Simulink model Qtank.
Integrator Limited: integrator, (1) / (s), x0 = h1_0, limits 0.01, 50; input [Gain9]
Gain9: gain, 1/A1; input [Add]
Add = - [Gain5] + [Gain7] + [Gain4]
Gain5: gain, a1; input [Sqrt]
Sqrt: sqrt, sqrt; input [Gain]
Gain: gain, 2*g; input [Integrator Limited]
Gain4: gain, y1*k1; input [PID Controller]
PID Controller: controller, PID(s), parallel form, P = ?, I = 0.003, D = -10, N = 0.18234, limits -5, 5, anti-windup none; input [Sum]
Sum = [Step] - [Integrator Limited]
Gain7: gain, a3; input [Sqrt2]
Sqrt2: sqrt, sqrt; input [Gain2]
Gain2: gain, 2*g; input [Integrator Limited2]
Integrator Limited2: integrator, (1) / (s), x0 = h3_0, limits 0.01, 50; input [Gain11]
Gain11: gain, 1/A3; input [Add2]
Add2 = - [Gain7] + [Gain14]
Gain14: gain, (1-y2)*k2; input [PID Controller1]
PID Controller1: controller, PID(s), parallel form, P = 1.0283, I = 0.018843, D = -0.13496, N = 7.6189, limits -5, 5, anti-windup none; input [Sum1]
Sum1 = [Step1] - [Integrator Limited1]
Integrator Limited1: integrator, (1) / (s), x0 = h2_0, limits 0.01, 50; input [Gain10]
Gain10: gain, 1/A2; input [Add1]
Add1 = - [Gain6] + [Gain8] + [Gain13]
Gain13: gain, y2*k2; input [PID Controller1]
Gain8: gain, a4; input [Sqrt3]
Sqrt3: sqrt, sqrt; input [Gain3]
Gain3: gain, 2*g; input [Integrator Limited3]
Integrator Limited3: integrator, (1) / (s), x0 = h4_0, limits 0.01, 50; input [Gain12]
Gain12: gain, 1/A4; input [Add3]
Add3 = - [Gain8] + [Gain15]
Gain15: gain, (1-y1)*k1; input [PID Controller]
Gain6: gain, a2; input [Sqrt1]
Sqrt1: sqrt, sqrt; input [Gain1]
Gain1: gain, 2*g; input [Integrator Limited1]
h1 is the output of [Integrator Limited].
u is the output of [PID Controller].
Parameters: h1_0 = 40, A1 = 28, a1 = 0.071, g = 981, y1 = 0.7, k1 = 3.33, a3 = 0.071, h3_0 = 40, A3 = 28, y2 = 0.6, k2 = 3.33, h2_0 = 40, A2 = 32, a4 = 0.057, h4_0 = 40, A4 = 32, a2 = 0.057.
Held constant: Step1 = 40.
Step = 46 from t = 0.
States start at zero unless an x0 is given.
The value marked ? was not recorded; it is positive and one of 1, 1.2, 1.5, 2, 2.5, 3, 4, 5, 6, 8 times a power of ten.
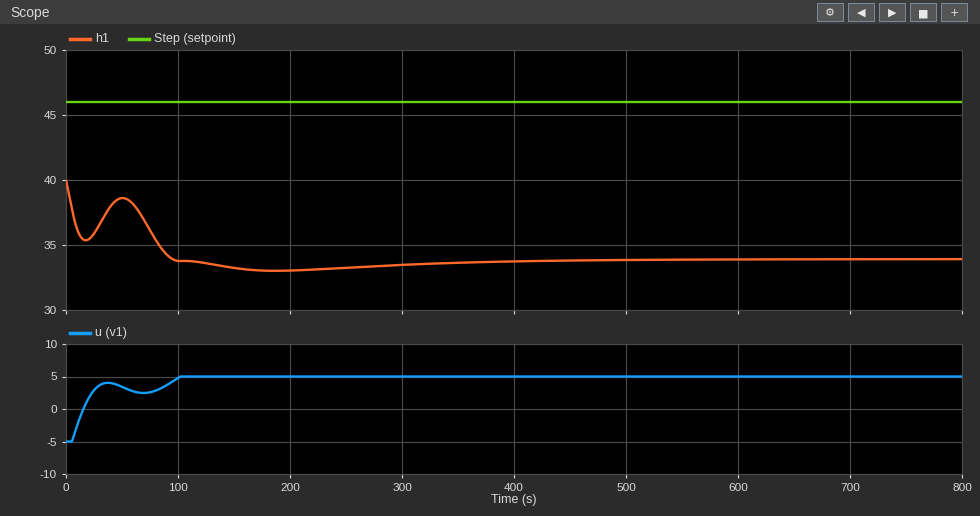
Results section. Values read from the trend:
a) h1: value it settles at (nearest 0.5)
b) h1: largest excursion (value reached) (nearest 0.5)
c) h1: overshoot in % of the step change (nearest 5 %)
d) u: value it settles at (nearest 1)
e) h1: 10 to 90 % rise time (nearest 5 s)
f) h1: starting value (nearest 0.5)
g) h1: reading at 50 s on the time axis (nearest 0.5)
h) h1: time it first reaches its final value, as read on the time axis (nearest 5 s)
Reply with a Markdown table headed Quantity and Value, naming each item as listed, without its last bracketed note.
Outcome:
| Quantity | Value |
|---|---|
| h1: value it settles at | 34.0 |
| h1: largest excursion (value reached) | 33.0 |
| h1: overshoot in % of the step change | 15 % |
| u: value it settles at | 5 |
| h1: 10 to 90 % rise time | 85 s |
| h1: starting value | 40.0 |
| h1: reading at 50 s on the time axis | 38.5 |
| h1: time it first reaches its final value, as read on the time axis | 95 s |
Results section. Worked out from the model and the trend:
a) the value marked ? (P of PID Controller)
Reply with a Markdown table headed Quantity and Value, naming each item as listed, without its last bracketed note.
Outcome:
| Quantity | Value |
|---|---|
| the value marked ? | 0.2 |
